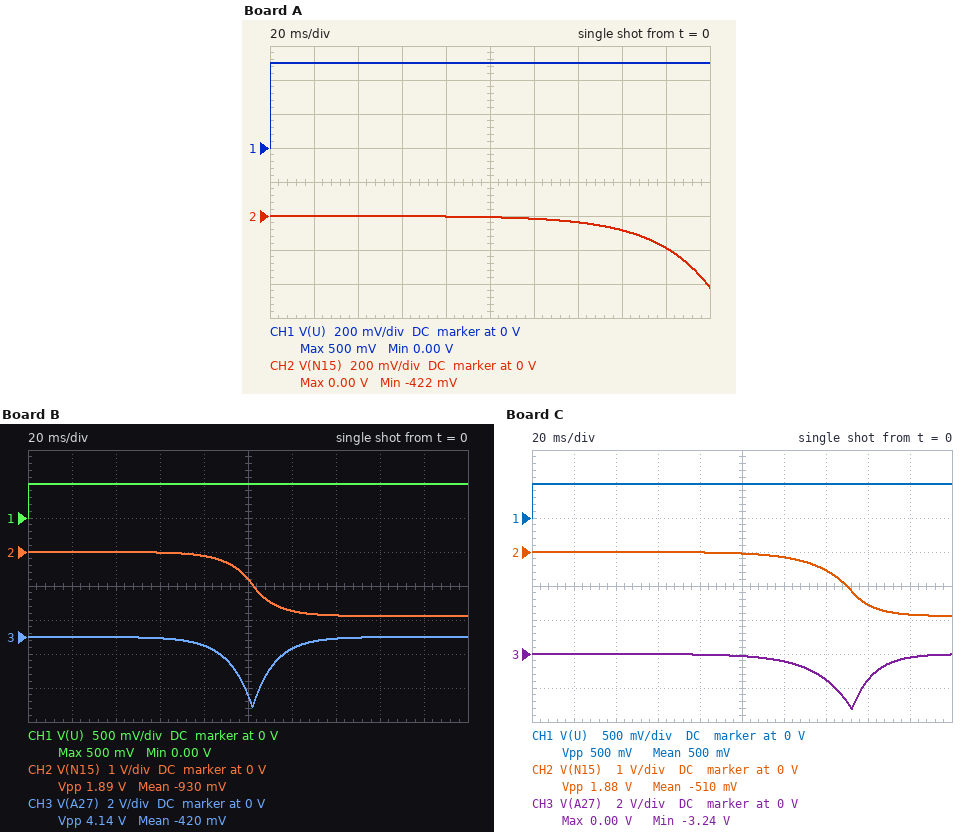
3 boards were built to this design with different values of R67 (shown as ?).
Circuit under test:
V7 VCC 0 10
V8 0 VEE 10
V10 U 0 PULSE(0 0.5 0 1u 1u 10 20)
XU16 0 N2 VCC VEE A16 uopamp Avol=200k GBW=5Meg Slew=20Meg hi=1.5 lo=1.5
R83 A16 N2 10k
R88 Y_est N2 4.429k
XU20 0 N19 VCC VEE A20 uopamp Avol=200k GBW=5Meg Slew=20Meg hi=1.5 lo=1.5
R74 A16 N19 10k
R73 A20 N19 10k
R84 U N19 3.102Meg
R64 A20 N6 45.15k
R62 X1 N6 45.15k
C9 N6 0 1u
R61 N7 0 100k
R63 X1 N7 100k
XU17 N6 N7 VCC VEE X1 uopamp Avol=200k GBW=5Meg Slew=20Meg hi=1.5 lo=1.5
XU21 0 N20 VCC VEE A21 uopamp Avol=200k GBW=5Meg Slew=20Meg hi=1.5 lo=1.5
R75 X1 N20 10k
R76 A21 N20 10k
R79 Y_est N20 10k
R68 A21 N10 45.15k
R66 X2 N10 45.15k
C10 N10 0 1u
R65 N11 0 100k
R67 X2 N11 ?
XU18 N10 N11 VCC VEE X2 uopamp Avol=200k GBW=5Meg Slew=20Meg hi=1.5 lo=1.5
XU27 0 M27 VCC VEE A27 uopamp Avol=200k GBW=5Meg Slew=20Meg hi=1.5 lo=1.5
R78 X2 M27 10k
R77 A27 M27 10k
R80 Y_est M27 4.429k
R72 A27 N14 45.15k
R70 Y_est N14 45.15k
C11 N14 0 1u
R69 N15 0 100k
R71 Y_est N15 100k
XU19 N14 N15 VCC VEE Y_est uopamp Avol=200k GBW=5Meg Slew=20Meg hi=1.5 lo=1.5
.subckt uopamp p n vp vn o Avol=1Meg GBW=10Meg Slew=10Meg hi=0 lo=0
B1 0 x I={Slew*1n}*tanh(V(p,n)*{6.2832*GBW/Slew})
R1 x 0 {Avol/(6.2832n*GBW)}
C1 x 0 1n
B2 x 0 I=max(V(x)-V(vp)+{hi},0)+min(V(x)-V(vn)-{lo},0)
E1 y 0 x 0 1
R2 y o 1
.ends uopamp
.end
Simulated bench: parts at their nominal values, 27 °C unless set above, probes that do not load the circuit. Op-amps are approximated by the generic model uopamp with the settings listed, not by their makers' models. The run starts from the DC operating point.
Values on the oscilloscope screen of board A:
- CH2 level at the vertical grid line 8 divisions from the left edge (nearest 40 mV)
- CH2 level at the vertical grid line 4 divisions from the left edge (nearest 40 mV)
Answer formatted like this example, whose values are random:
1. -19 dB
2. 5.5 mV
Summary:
1. -80 mV
2. 0 V
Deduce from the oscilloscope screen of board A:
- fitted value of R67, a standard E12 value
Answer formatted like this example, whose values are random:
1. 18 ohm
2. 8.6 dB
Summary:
1. 82 kΩ
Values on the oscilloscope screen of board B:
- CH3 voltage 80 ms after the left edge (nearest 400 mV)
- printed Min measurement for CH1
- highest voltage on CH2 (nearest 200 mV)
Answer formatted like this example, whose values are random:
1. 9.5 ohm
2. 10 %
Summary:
1. -400 mV
2. 0.00 V
3. 0 V
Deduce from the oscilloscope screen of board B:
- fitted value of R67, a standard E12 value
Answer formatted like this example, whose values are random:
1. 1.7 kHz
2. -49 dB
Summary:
1. 330 kΩ
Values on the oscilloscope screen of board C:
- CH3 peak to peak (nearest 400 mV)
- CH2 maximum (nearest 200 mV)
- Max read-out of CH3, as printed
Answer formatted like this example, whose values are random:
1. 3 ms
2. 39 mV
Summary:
1. 3.2 V
2. 0 V
3. 0.00 V
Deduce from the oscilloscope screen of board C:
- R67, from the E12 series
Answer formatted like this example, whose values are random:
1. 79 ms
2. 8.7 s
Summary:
1. 180 kΩ
